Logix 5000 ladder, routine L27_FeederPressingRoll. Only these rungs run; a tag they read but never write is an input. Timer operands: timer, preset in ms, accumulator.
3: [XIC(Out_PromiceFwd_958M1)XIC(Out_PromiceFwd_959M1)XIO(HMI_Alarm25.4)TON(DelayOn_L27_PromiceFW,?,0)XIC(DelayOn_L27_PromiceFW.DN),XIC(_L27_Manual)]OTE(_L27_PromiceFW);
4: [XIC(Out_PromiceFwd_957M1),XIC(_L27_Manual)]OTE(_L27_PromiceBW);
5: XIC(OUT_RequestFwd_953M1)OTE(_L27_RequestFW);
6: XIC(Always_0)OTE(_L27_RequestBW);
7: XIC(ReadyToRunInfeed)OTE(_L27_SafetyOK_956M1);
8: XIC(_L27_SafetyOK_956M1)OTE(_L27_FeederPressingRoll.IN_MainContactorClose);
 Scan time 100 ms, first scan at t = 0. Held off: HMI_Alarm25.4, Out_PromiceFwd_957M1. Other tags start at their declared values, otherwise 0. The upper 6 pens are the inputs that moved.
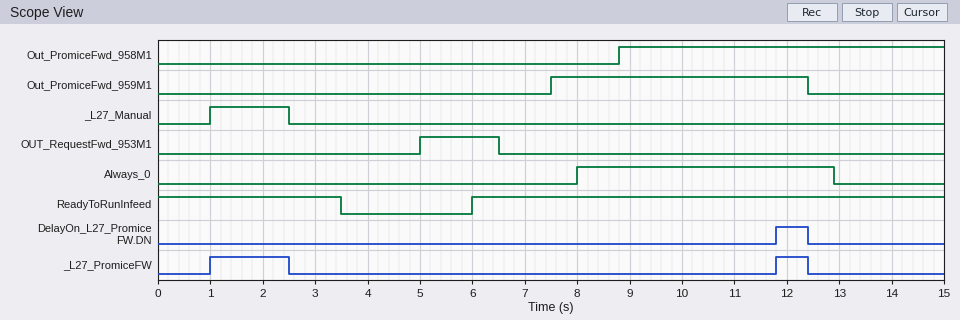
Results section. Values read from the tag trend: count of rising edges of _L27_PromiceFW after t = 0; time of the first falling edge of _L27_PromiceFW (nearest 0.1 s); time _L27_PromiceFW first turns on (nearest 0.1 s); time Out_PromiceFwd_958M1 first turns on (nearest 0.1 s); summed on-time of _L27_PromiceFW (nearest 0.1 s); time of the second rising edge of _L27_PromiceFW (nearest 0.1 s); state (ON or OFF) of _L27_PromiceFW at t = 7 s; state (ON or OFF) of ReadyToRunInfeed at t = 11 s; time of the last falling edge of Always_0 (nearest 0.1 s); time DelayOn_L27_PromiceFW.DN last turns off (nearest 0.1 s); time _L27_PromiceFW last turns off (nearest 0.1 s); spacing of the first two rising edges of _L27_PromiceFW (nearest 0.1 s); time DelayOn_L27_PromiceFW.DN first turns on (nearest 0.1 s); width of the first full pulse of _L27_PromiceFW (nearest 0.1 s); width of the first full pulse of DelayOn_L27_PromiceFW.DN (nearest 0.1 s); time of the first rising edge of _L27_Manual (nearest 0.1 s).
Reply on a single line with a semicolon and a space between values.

2; 2.5 s; 1.0 s; 8.8 s; 2.1 s; 11.8 s; OFF; ON; 12.9 s; 12.4 s; 12.4 s; 10.8 s; 11.8 s; 1.5 s; 0.6 s; 1.0 s
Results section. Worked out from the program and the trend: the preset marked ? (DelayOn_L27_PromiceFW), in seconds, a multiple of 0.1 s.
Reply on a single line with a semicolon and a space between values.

3.0 s
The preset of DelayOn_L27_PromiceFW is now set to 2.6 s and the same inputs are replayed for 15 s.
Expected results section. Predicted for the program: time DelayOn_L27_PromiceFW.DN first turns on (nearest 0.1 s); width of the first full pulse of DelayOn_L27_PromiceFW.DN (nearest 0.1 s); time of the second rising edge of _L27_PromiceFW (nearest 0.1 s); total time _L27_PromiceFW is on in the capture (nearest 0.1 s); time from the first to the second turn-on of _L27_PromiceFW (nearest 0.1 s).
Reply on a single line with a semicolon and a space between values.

11.4 s; 1.0 s; 11.4 s; 2.5 s; 10.4 s
